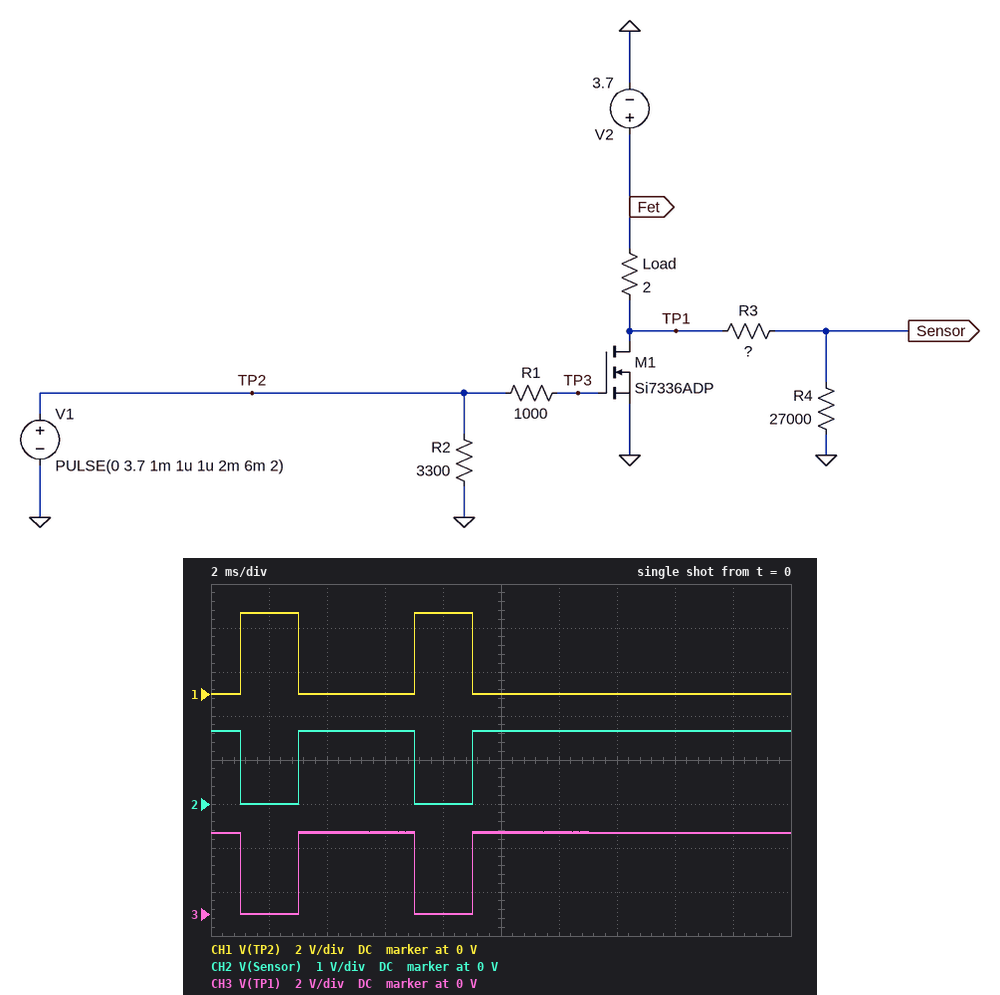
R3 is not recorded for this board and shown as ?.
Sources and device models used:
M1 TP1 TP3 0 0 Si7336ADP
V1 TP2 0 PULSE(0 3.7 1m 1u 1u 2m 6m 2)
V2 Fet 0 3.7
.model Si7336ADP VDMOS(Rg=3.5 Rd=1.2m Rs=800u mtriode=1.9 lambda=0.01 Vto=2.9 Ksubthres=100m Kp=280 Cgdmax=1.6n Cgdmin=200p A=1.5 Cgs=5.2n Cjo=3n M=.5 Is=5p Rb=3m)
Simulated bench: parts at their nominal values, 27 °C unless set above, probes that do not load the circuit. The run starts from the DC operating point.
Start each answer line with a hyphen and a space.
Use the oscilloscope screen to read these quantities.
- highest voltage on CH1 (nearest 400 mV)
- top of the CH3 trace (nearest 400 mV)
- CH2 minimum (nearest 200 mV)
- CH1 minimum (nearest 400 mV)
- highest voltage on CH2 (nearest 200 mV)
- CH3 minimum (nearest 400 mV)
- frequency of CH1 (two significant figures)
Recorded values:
- 3.6 V
- 3.6 V
- 0 V
- 0 V
- 1.6 V
- 0 V
- 170 Hz
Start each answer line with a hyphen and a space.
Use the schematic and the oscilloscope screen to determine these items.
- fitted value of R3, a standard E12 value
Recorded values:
- 33 kΩ
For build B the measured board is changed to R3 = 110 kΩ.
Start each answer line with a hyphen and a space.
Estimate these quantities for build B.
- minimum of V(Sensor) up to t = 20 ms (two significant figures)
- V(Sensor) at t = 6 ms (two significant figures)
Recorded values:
- 1.6 mV
- 730 mV
